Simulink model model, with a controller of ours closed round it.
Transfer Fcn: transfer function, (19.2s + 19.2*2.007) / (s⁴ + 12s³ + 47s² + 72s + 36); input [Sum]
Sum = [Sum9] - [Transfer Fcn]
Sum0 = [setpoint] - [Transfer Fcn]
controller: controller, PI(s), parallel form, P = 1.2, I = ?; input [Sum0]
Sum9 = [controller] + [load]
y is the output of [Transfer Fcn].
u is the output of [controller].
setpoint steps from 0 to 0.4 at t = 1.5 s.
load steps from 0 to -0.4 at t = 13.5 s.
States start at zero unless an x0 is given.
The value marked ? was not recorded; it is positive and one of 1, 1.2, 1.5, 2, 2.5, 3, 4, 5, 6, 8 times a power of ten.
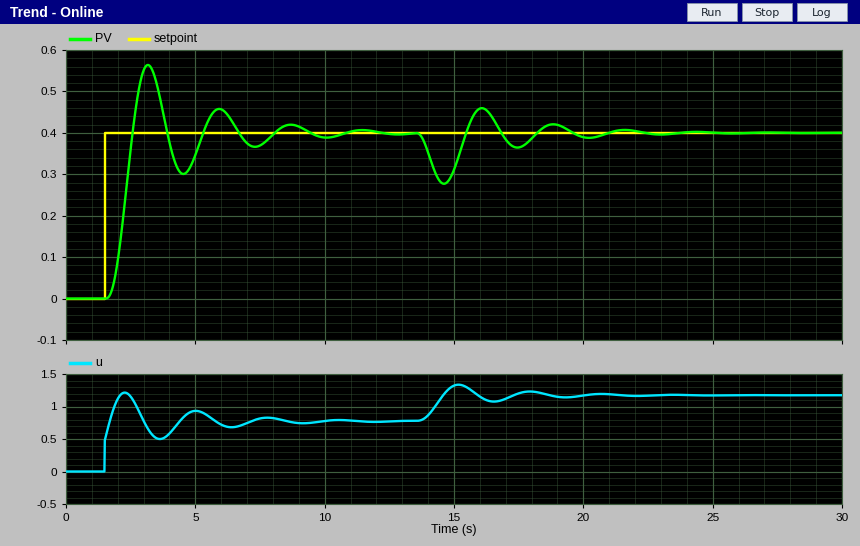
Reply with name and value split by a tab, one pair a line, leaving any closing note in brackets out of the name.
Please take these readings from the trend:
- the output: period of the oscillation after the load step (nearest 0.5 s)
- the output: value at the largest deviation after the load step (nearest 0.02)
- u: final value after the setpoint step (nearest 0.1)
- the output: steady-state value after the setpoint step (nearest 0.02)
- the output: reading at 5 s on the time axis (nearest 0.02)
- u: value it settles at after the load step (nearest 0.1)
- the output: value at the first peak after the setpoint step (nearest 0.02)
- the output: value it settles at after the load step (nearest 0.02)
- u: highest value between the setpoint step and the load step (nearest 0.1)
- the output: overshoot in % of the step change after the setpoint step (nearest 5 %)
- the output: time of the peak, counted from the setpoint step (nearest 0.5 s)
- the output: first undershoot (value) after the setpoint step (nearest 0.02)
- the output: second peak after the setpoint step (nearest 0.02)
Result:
the output: period of the oscillation after the load step	3.0 s
the output: value at the largest deviation after the load step	0.28
u: final value after the setpoint step	0.8
the output: steady-state value after the setpoint step	0.40
the output: reading at 5 s on the time axis	0.34
u: value it settles at after the load step	1.2
the output: value at the first peak after the setpoint step	0.56
the output: value it settles at after the load step	0.40
u: highest value between the setpoint step and the load step	1.2
the output: overshoot in % of the step change after the setpoint step	40 %
the output: time of the peak, counted from the setpoint step	1.5 s
the output: first undershoot (value) after the setpoint step	0.30
the output: second peak after the setpoint step	0.46
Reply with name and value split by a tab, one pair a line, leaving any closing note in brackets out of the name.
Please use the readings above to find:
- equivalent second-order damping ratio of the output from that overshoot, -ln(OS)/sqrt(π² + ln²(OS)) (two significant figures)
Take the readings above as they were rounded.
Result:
equivalent second-order damping ratio of the output from that overshoot, -ln(OS)/sqrt(π² + ln²(OS))	0.28
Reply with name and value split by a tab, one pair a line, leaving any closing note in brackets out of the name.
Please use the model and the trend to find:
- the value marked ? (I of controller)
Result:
the value marked ?	4
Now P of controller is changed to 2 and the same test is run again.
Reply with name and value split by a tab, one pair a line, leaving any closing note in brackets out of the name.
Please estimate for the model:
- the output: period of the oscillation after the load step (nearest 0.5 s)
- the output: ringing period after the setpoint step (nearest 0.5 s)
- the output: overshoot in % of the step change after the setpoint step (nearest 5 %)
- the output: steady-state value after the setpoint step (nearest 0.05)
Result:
the output: period of the oscillation after the load step	2.5 s
the output: ringing period after the setpoint step	2.5 s
the output: overshoot in % of the step change after the setpoint step	35 %
the output: steady-state value after the setpoint step	0.40
